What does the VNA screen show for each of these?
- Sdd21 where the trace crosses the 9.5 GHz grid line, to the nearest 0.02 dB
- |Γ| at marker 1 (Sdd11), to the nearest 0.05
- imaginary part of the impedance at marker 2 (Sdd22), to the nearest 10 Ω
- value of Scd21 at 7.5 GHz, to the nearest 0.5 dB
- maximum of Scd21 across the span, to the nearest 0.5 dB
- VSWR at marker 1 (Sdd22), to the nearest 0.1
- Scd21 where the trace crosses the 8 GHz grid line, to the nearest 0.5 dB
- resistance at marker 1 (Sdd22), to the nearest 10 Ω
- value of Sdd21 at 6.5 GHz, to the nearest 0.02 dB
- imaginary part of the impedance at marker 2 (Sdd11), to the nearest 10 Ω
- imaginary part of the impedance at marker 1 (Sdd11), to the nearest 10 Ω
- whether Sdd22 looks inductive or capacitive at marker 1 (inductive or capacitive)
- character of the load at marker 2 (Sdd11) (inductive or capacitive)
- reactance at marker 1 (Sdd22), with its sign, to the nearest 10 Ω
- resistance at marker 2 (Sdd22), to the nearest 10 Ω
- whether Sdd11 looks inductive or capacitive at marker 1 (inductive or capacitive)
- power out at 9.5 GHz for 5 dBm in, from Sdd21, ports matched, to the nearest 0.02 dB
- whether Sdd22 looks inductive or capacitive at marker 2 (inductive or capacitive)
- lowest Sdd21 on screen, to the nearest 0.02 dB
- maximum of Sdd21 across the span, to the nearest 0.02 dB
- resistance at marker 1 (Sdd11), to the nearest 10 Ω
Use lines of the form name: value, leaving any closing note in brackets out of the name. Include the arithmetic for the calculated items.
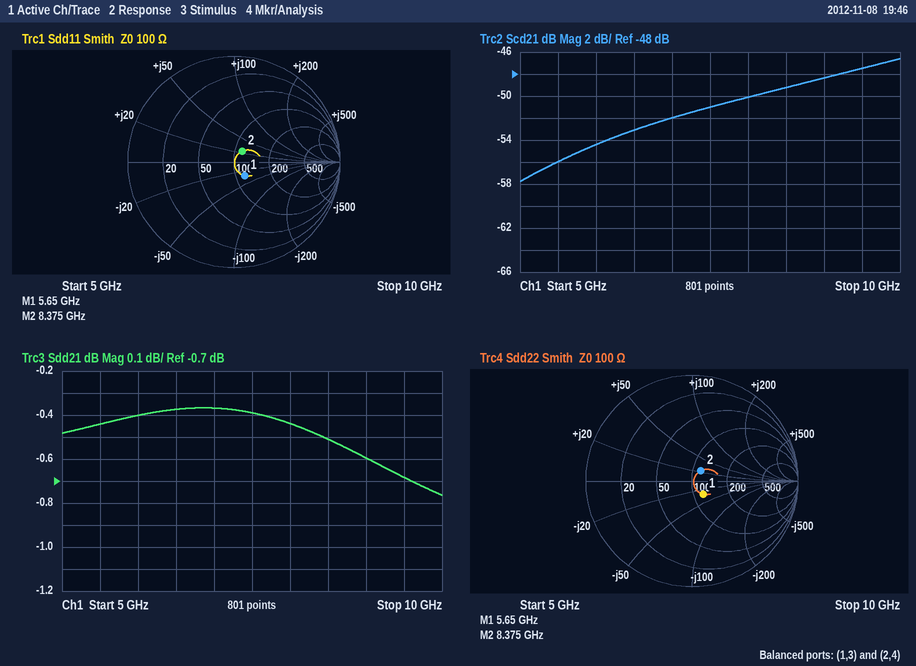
Sdd21 where the trace crosses the 9.5 GHz grid line, to the nearest 0.02 dB: -0.68 dB
|Γ| at marker 1 (Sdd11), to the nearest 0.05: 0.15
imaginary part of the impedance at marker 2 (Sdd22), to the nearest 10 Ω: +20 Ω
value of Scd21 at 7.5 GHz, to the nearest 0.5 dB: -51.0 dB
maximum of Scd21 across the span, to the nearest 0.5 dB: -46.5 dB
VSWR at marker 1 (Sdd22), to the nearest 0.1: 1.4
Scd21 where the trace crosses the 8 GHz grid line, to the nearest 0.5 dB: -50.0 dB
resistance at marker 1 (Sdd22), to the nearest 10 Ω: 120 Ω
value of Sdd21 at 6.5 GHz, to the nearest 0.02 dB: -0.38 dB
imaginary part of the impedance at marker 2 (Sdd11), to the nearest 10 Ω: +20 Ω
imaginary part of the impedance at marker 1 (Sdd11), to the nearest 10 Ω: -30 Ω
whether Sdd22 looks inductive or capacitive at marker 1: capacitive
character of the load at marker 2 (Sdd11): inductive
reactance at marker 1 (Sdd22), with its sign, to the nearest 10 Ω: -30 Ω
resistance at marker 2 (Sdd22), to the nearest 10 Ω: 120 Ω
whether Sdd11 looks inductive or capacitive at marker 1: capacitive
power out at 9.5 GHz for 5 dBm in, from Sdd21, ports matched, to the nearest 0.02 dB: 5 dBm + (-0.68 dB) = 4.32 dBm
whether Sdd22 looks inductive or capacitive at marker 2: inductive
lowest Sdd21 on screen, to the nearest 0.02 dB: -0.76 dB
maximum of Sdd21 across the span, to the nearest 0.02 dB: -0.36 dB
resistance at marker 1 (Sdd11), to the nearest 10 Ω: 120 Ω
